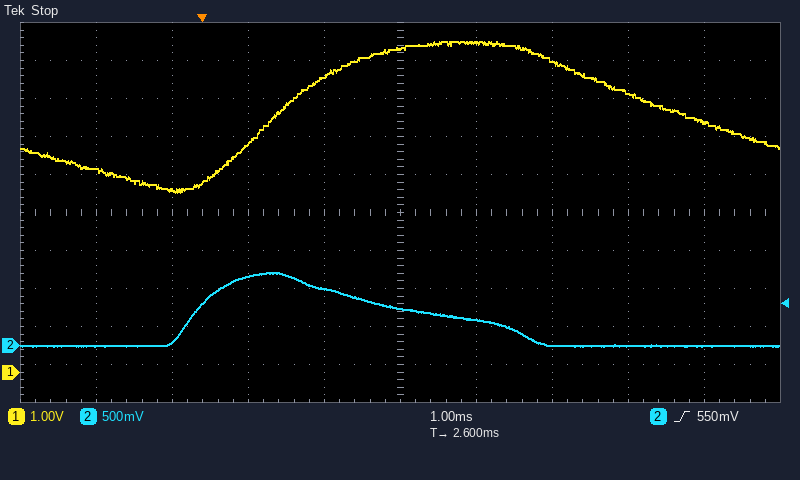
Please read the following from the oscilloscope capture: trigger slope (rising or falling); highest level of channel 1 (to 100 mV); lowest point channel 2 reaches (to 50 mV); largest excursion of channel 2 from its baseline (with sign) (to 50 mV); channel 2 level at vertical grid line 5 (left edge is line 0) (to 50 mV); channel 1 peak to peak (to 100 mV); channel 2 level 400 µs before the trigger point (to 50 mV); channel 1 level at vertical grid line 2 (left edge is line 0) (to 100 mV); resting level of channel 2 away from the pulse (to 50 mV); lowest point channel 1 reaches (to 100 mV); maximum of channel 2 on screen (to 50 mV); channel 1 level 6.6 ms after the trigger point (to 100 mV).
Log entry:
rising
8.7 V
0 mV
+950 mV
500 mV
4.0 V
50 mV
4.8 V
0 mV
4.7 V
950 mV
6.6 V
